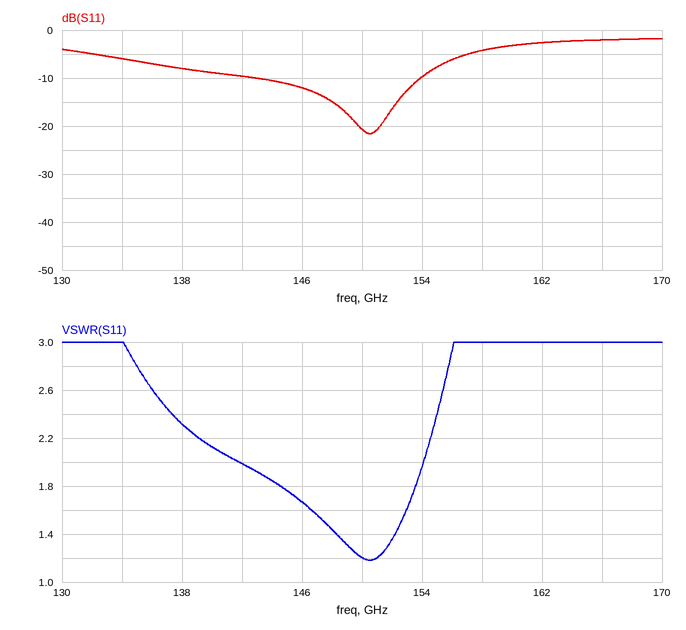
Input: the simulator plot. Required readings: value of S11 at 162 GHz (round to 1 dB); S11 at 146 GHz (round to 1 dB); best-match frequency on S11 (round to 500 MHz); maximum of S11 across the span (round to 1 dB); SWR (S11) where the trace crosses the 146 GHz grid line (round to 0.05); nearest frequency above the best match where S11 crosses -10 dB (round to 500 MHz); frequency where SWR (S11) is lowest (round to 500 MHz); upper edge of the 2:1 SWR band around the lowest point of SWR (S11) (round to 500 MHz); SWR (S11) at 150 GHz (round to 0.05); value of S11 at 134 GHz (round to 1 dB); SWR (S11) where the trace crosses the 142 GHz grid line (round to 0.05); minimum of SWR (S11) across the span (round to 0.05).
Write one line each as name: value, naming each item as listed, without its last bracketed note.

value of S11 at 162 GHz: -3 dB
S11 at 146 GHz: -12 dB
best-match frequency on S11: 150.5 GHz
maximum of S11 across the span: -2 dB
SWR (S11) where the trace crosses the 146 GHz grid line: 1.65
nearest frequency above the best match where S11 crosses -10 dB: 154.0 GHz
frequency where SWR (S11) is lowest: 150.5 GHz
upper edge of the 2:1 SWR band around the lowest point of SWR (S11): 154.0 GHz
SWR (S11) at 150 GHz: 1.20
value of S11 at 134 GHz: -6 dB
SWR (S11) where the trace crosses the 142 GHz grid line: 2.00
minimum of SWR (S11) across the span: 1.20
